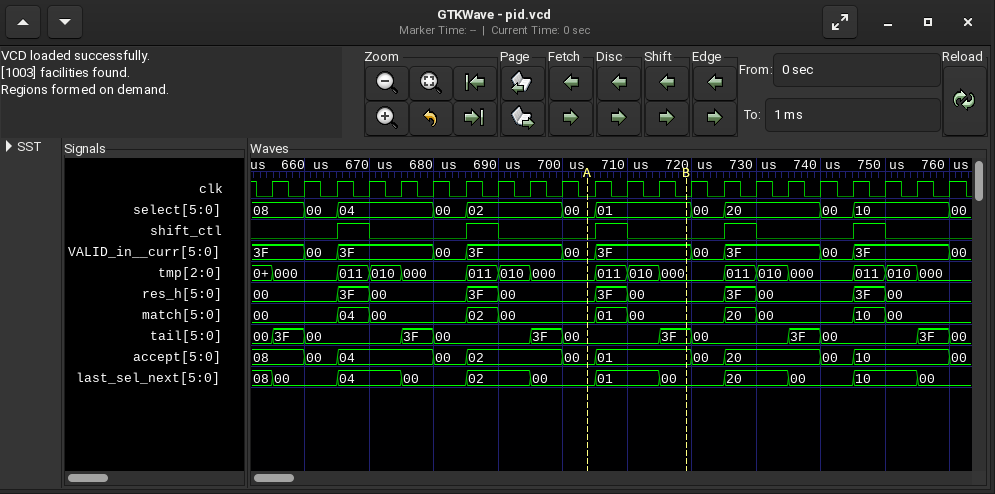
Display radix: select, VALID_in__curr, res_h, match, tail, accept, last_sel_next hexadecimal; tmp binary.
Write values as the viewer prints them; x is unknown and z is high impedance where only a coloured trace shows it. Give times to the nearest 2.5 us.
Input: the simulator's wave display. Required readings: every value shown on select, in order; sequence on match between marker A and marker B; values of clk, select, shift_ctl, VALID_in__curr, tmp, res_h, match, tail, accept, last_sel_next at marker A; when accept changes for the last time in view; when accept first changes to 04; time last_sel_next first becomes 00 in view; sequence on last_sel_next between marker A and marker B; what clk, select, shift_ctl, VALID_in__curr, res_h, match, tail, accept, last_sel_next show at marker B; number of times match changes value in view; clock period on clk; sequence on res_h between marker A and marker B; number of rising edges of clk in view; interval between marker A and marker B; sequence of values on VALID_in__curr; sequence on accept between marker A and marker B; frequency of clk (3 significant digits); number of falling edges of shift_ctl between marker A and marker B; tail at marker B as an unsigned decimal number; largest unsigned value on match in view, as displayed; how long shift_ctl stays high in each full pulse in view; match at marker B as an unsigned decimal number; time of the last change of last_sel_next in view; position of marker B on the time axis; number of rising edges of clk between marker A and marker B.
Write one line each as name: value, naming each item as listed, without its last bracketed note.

every value shown on select, in order: 08, 00, 04, 00, 02, 00, 01, 00, 20, 00, 10, 00
sequence on match between marker A and marker B: 00, 01, 00
values of clk, select, shift_ctl, VALID_in__curr, tmp, res_h, match, tail, accept, last_sel_next at marker A: clk=0, select=00, shift_ctl=0, VALID_in__curr=00, tmp=000, res_h=00, match=00, tail=00, accept=00, last_sel_next=00
when accept changes for the last time in view: 760 us
when accept first changes to 04: 665 us
time last_sel_next first becomes 00 in view: 655 us
sequence on last_sel_next between marker A and marker B: 00, 01, 00
what clk, select, shift_ctl, VALID_in__curr, res_h, match, tail, accept, last_sel_next show at marker B: clk=0, select=01, shift_ctl=0, VALID_in__curr=3F, res_h=00, match=00, tail=3F, accept=01, last_sel_next=00
number of times match changes value in view: 10
clock period on clk: 5 us
sequence on res_h between marker A and marker B: 00, 3F, 00
number of rising edges of clk in view: 22
interval between marker A and marker B: 15 us
sequence of values on VALID_in__curr: 3F, 00, 3F, 00, 3F, 00, 3F, 00, 3F, 00, 3F, 00
sequence on accept between marker A and marker B: 00, 01
frequency of clk: 200 kHz
number of falling edges of shift_ctl between marker A and marker B: 1
tail at marker B as an unsigned decimal number: 63
largest unsigned value on match in view, as displayed: 20
how long shift_ctl stays high in each full pulse in view: 5 us, 5 us, 5 us, 5 us, 5 us
match at marker B as an unsigned decimal number: 0
time of the last change of last_sel_next in view: 755 us
position of marker B on the time axis: 720 us
number of rising edges of clk between marker A and marker B: 3
